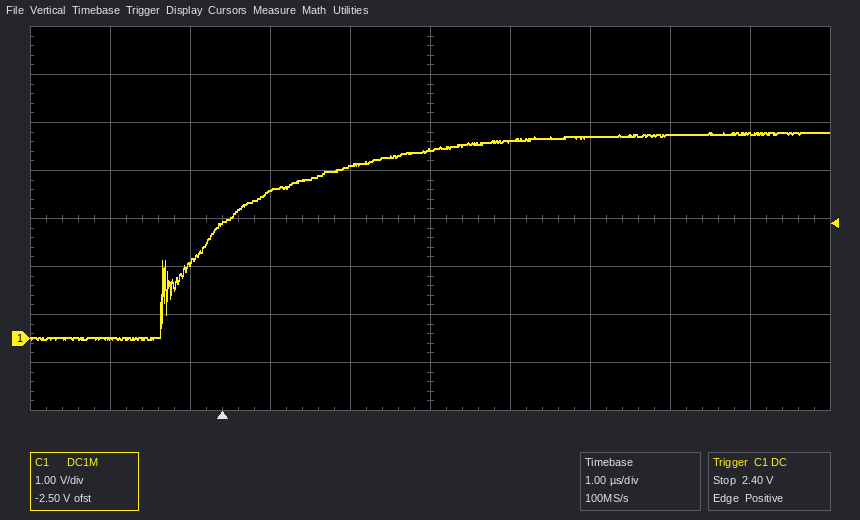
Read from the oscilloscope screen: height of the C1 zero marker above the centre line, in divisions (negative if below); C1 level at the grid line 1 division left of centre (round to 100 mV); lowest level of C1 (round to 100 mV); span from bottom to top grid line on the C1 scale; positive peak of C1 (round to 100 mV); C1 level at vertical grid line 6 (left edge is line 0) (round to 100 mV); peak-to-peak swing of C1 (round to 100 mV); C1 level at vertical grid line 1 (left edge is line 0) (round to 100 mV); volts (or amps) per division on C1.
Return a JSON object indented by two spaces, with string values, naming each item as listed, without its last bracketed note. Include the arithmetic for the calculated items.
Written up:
{
  "height of the C1 zero marker above the centre line, in divisions": "-2.5 div",
  "C1 level at the grid line 1 division left of centre": "3.6 V",
  "lowest level of C1": "0.0 V",
  "span from bottom to top grid line on the C1 scale": "8 V",
  "positive peak of C1": "4.3 V",
  "C1 level at vertical grid line 6 (left edge is line 0)": "4.1 V",
  "peak-to-peak swing of C1": "4.3 V − (0.0 V) = 4.3 V",
  "C1 level at vertical grid line 1 (left edge is line 0)": "0.0 V",
  "volts (or amps) per division on C1": "1 V"
}
